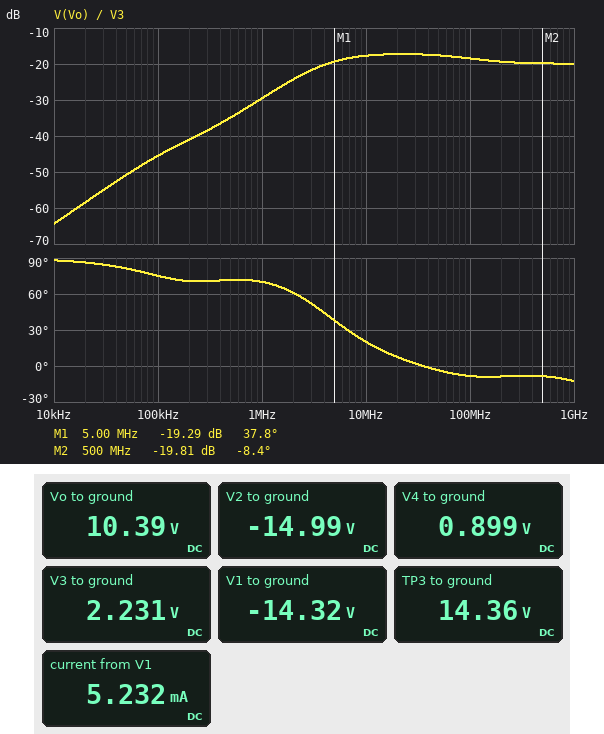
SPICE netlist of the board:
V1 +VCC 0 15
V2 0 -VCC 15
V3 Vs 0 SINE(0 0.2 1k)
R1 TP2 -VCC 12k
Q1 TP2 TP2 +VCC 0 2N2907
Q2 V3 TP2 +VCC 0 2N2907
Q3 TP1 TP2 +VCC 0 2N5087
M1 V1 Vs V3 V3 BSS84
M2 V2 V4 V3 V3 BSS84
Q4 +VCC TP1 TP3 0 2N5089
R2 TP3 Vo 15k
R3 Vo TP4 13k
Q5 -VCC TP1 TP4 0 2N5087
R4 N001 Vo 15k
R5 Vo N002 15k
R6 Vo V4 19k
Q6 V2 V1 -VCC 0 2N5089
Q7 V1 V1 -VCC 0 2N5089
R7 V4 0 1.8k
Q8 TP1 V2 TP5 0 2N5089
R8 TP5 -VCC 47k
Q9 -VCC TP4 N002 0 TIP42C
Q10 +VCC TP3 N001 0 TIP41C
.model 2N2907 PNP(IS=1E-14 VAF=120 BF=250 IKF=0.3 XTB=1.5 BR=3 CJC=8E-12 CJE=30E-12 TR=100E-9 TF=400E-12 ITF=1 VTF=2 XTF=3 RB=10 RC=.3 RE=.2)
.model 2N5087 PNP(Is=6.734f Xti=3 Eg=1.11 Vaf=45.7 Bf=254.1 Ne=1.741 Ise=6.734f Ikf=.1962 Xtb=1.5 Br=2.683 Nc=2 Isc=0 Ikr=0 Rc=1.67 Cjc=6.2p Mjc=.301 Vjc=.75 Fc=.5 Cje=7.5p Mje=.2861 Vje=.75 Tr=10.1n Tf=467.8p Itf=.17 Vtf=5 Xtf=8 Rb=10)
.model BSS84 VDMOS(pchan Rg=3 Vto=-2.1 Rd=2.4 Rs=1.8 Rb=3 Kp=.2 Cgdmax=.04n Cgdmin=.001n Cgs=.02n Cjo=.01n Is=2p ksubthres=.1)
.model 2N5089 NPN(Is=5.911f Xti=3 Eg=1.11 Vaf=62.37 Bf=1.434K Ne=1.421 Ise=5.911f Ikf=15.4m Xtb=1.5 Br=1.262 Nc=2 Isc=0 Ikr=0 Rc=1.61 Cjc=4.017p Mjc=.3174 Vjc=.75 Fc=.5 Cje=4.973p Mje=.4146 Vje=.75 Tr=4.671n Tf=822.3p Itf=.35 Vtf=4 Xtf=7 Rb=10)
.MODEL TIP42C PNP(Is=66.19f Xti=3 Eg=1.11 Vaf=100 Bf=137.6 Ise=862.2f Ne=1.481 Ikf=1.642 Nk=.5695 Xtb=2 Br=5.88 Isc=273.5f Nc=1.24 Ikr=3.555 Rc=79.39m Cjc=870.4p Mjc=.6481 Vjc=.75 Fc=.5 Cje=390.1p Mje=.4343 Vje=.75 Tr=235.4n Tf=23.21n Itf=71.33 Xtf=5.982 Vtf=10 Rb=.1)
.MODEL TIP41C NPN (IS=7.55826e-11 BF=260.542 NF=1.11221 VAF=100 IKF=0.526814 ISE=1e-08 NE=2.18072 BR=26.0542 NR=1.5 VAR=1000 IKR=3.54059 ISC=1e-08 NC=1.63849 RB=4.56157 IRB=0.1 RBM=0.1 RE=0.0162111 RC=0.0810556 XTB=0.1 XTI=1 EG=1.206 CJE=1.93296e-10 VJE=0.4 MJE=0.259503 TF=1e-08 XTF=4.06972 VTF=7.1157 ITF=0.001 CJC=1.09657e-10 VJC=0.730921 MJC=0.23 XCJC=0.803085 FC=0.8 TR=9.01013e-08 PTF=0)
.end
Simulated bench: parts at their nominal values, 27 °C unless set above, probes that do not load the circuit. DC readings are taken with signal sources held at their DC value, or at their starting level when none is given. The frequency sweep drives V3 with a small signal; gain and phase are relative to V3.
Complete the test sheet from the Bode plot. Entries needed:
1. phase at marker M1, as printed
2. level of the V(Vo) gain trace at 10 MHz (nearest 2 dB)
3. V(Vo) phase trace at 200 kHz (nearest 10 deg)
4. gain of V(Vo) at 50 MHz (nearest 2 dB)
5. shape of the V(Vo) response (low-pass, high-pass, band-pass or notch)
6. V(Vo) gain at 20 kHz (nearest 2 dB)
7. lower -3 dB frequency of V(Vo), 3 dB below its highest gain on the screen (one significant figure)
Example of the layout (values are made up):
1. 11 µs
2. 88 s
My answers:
1. 37.8 deg
2. -18 dB
3. 70 deg
4. -18 dB
5. high-pass
6. -58 dB
7. 4 MHz
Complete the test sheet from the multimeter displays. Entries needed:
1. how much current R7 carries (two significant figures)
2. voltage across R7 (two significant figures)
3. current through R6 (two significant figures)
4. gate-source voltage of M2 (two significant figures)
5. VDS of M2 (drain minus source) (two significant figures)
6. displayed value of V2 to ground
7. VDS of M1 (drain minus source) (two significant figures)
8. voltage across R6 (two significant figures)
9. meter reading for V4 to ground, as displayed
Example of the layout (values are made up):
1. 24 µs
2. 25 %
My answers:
1. 500 µA
2. 900 mV
3. 500 µA
4. -1.3 V
5. -17 V
6. -14.99 V
7. -17 V
8. 9.5 V
9. 0.899 V
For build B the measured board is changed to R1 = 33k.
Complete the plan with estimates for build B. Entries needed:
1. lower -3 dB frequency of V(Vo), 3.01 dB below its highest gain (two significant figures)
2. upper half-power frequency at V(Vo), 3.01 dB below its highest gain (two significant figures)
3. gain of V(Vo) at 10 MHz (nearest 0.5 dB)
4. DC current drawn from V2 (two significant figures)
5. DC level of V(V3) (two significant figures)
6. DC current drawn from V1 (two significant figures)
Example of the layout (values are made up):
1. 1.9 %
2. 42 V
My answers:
1. 3.7 MHz
2. 2.5 GHz
3. -18.0 dB
4. 1.7 mA
5. 2.1 V
6. 2.2 mA
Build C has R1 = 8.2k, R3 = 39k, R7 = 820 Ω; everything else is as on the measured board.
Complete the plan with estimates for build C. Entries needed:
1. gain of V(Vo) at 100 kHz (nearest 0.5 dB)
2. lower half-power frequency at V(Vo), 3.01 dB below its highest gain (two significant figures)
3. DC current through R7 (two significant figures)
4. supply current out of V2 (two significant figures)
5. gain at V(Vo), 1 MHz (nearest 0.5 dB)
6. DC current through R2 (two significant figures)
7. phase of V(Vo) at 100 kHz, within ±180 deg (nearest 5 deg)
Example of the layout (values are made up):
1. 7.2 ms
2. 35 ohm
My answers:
1. -52.0 dB
2. 7.8 MHz
3. 520 µA
4. 6.9 mA
5. -34.5 dB
6. 270 µA
7. 80 deg
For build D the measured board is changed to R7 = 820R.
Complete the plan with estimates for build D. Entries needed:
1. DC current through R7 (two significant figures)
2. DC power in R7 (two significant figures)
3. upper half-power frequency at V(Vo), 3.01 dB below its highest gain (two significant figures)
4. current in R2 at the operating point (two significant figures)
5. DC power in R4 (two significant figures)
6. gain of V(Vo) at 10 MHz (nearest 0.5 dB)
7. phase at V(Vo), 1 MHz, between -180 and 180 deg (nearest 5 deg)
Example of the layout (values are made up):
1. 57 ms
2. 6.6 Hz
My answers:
1. 520 µA
2. 220 µW
3. 2.1 GHz
4. 270 µA
5. 900 µW
6. -19.5 dB
7. 75 deg
